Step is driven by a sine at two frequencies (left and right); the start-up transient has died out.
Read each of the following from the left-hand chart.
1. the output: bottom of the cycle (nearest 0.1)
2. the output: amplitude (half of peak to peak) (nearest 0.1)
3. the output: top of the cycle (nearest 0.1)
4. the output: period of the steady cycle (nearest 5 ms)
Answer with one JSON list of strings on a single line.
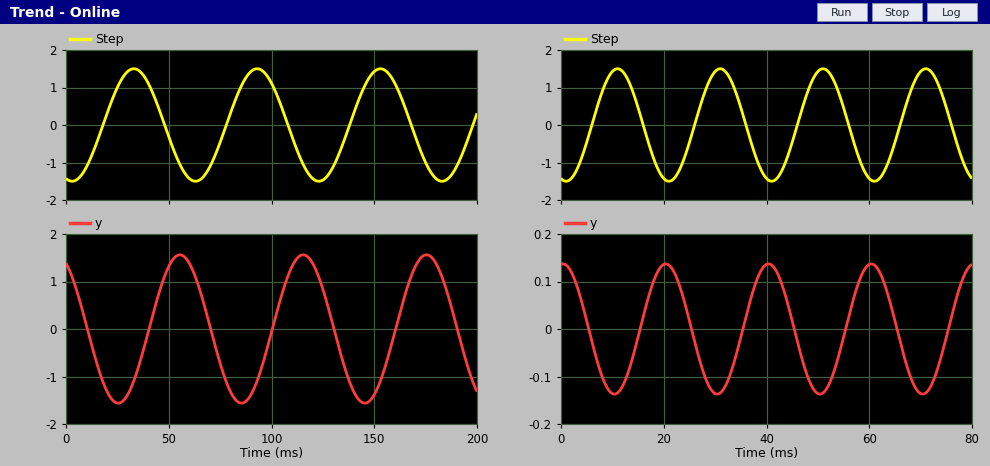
["-1.6", "1.6", "1.6", "60 ms"]
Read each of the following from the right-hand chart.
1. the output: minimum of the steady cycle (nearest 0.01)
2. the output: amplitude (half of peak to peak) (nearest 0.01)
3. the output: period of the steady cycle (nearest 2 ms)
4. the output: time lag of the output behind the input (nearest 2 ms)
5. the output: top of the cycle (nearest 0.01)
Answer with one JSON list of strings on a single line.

["-0.14", "0.14", "20 ms", "10 ms", "0.14"]
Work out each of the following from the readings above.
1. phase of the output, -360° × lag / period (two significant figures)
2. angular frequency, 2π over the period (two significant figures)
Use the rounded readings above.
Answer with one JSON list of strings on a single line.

["-180°", "0.31 rad/ms"]
